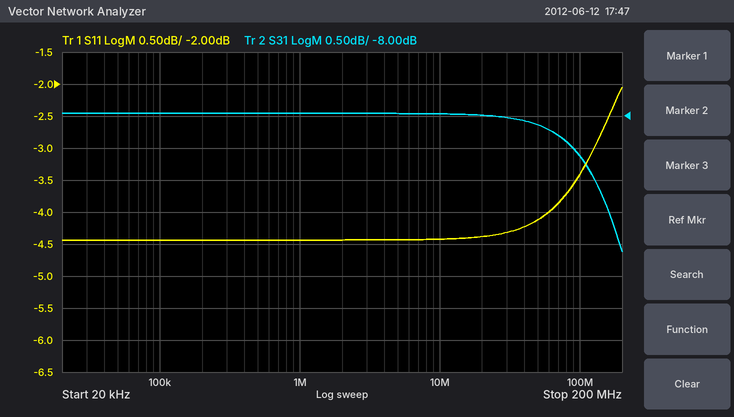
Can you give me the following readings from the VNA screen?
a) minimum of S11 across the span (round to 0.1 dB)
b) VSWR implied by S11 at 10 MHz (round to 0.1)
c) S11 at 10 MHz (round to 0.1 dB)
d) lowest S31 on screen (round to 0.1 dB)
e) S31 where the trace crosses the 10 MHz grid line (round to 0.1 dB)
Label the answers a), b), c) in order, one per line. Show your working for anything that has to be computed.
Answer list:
a) -4.4 dB
b) |Γ| = 10^(-4.4/20) = 0.6026; VSWR = (1 + 0.6026)/(1 − 0.6026) ≈ 4.0
c) -4.4 dB
d) -10.1 dB
e) -8.0 dB
